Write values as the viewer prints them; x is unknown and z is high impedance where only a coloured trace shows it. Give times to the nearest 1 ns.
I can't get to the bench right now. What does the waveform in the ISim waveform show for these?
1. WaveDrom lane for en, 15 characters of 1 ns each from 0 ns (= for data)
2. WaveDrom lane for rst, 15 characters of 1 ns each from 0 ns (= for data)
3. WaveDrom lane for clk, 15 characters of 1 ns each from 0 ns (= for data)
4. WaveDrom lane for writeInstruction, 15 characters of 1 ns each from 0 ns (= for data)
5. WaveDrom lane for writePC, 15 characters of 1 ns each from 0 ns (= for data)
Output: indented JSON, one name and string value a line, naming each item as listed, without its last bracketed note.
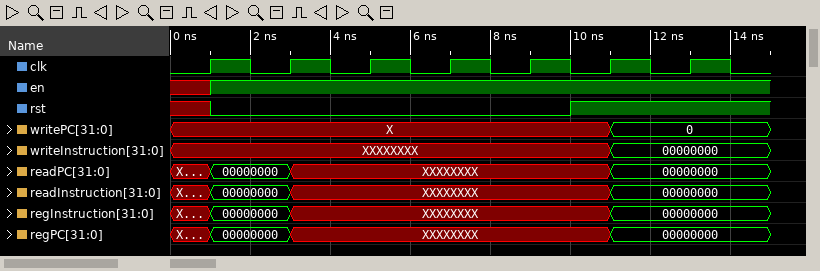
{
  "WaveDrom lane for en, 15 characters of 1 ns each from 0 ns": "{name: 'en', wave: 'x1.............'}",
  "WaveDrom lane for rst, 15 characters of 1 ns each from 0 ns": "{name: 'rst', wave: 'x0........1....'}",
  "WaveDrom lane for clk, 15 characters of 1 ns each from 0 ns": "{name: 'clk', wave: '010101010101010'}",
  "WaveDrom lane for writeInstruction, 15 characters of 1 ns each from 0 ns": "{name: 'writeInstruction', wave: 'x..........=...', data: '00000000'}",
  "WaveDrom lane for writePC, 15 characters of 1 ns each from 0 ns": "{name: 'writePC', wave: 'x..........=...', data: '0'}"
}
